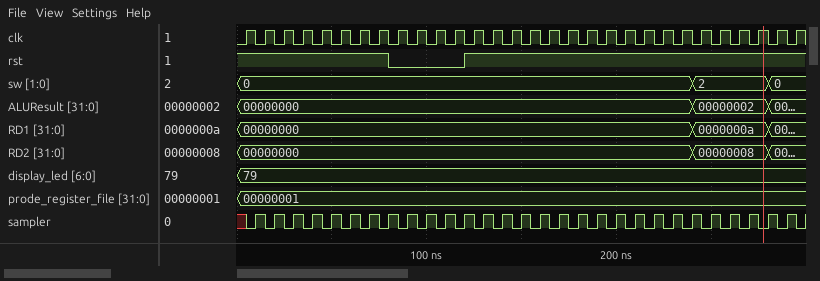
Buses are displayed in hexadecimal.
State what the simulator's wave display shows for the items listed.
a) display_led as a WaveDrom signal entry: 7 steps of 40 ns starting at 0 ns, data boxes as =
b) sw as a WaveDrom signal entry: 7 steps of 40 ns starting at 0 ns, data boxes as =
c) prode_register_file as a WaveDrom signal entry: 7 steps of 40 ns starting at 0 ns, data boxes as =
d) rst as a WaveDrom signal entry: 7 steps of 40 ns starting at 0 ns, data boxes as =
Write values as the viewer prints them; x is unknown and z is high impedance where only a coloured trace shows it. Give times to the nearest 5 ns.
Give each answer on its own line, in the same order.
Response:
{name: 'display_led', wave: '=......', data: '79'}
{name: 'sw', wave: '=.....=', data: '0 2'}
{name: 'prode_register_file', wave: '=......', data: '00000001'}
{name: 'rst', wave: '1.01...'}
